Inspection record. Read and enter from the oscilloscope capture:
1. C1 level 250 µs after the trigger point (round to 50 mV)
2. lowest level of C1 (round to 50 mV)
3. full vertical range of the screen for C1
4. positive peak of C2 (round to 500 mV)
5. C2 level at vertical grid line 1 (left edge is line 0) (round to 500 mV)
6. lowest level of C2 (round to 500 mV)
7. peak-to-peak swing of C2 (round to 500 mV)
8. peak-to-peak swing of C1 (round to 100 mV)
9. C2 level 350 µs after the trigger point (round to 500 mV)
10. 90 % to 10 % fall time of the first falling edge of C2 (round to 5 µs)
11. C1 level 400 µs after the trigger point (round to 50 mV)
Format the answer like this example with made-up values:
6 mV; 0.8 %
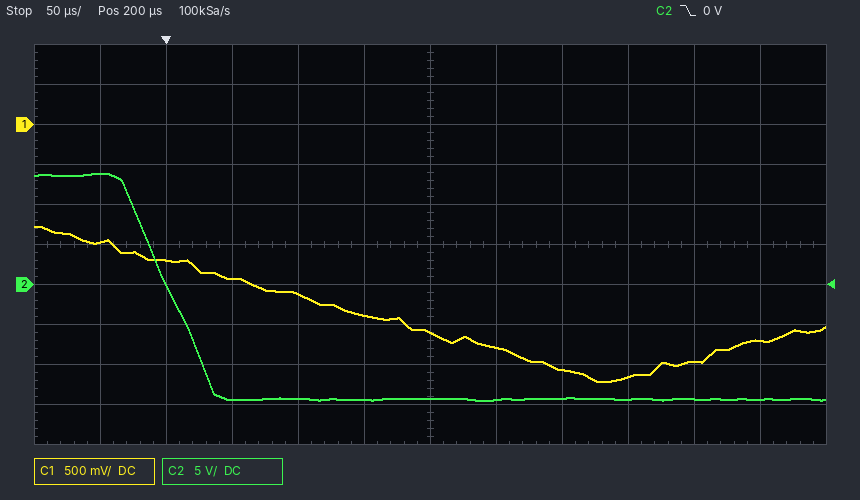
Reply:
-2.80 V; -3.20 V; 5 V; 14.0 V; 14.0 V; -14.5 V; 28.5 V; 1.90 V; -14.5 V; 60 µs; -2.95 V
